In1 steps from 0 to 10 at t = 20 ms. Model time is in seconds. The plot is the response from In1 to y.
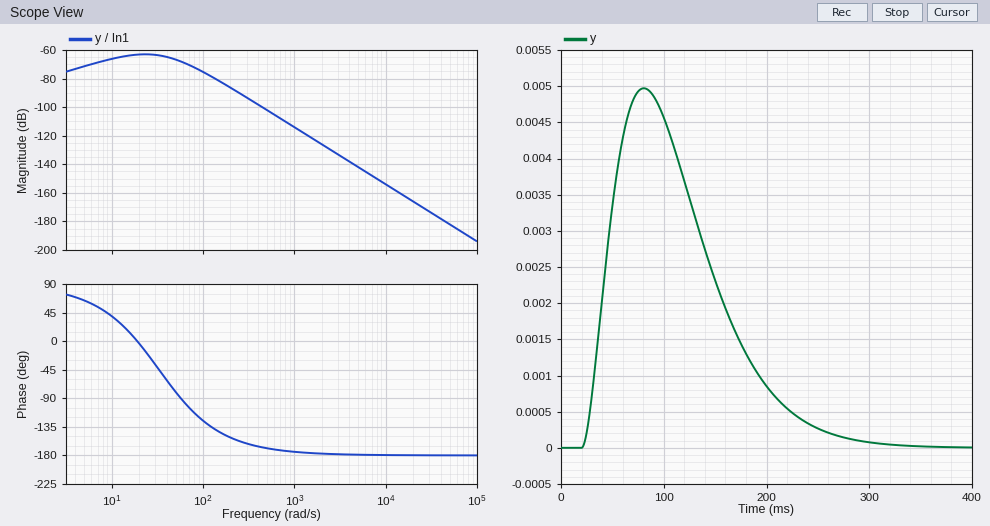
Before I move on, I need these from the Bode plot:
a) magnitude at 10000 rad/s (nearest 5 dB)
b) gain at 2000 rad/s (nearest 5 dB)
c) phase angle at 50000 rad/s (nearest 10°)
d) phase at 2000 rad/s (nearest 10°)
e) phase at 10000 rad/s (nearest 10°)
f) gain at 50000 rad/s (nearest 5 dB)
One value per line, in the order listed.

-155 dB
-125 dB
-180°
-180°
-180°
-180 dB
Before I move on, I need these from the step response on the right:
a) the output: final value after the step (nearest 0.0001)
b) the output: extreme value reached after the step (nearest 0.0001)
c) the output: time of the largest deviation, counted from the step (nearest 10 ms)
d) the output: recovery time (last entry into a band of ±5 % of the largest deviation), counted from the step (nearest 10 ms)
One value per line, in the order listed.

0.0000
0.0050
60 ms
230 ms
